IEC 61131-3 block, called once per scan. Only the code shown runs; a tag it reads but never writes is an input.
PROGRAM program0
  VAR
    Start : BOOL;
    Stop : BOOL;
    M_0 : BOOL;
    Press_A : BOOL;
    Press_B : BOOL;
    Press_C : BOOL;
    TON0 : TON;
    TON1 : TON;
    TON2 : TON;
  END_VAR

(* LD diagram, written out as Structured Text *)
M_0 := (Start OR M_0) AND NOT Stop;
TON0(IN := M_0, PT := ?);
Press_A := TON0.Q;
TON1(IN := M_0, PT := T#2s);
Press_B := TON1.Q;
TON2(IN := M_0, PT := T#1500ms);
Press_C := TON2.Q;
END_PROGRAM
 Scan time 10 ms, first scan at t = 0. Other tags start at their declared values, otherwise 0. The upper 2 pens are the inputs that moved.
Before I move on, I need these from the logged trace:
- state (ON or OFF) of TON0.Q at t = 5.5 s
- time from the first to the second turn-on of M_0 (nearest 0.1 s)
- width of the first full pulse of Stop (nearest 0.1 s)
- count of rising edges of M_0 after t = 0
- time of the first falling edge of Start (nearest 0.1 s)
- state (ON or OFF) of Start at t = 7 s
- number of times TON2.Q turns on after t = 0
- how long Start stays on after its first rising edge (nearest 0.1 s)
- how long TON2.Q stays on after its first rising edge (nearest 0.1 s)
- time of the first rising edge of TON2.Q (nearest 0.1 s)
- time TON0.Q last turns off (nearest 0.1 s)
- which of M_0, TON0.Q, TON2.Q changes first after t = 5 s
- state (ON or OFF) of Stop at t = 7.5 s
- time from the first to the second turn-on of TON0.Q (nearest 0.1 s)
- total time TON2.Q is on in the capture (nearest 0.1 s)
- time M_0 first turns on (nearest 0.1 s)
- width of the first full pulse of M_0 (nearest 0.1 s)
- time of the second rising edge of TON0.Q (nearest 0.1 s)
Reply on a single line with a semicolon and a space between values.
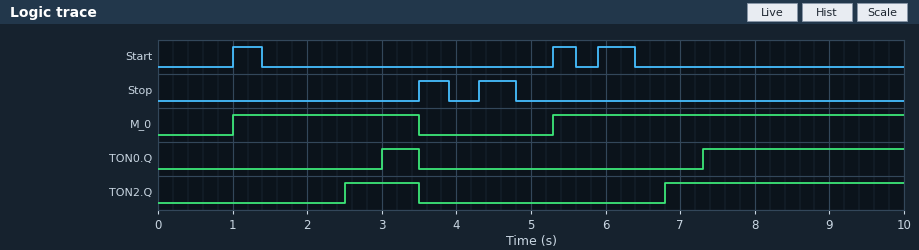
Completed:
OFF; 4.3 s; 0.4 s; 2; 1.4 s; OFF; 2; 0.4 s; 1.0 s; 2.5 s; 3.5 s; M_0; OFF; 4.3 s; 4.2 s; 1.0 s; 2.5 s; 7.3 s
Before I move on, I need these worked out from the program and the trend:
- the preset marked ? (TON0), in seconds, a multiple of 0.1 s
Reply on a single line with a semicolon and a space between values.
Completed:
2.0 s
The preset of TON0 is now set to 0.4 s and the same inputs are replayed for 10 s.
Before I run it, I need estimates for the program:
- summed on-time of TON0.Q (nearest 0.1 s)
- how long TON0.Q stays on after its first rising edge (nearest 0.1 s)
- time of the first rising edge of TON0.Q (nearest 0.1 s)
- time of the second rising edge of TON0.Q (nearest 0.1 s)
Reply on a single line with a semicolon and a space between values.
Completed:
6.4 s; 2.1 s; 1.4 s; 5.7 s
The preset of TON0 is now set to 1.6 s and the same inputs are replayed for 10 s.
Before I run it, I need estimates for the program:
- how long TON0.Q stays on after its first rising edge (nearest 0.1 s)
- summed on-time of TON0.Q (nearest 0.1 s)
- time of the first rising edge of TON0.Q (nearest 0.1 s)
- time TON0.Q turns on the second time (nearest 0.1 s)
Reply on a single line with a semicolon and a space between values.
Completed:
0.9 s; 4.0 s; 2.6 s; 6.9 s
